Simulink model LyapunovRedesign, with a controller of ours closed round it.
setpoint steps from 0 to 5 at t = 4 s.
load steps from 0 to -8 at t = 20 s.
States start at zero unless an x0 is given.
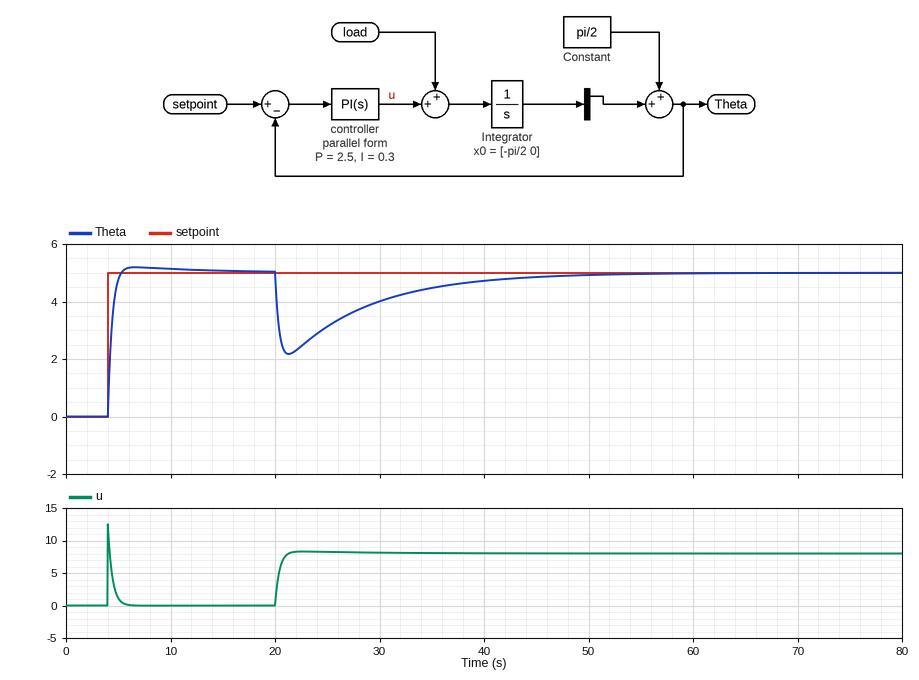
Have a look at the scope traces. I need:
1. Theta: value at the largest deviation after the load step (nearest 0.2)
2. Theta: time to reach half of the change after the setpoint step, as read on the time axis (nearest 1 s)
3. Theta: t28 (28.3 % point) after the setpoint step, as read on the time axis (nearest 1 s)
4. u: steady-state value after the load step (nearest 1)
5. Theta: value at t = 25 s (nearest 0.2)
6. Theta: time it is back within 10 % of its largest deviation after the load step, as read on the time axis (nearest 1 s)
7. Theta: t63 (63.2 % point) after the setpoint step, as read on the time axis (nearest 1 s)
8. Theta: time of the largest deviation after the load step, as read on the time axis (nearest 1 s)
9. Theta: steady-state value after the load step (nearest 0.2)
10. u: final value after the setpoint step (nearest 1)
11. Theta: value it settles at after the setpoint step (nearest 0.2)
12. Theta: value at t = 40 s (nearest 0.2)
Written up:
2.2
4 s
4 s
8
3.2
40 s
4 s
21 s
5.0
0
5.0
4.8
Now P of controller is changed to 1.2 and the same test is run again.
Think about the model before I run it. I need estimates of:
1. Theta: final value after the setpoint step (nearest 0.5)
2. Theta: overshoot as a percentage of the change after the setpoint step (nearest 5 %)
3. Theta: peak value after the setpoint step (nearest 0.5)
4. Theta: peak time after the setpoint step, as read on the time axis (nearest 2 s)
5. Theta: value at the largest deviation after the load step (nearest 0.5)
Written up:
5.0
10 %
5.5
8 s
0.0
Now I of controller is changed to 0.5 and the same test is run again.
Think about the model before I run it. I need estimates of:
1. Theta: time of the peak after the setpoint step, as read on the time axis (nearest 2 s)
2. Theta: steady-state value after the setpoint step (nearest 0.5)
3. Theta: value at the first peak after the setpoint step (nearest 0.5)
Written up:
6 s
5.0
5.5
